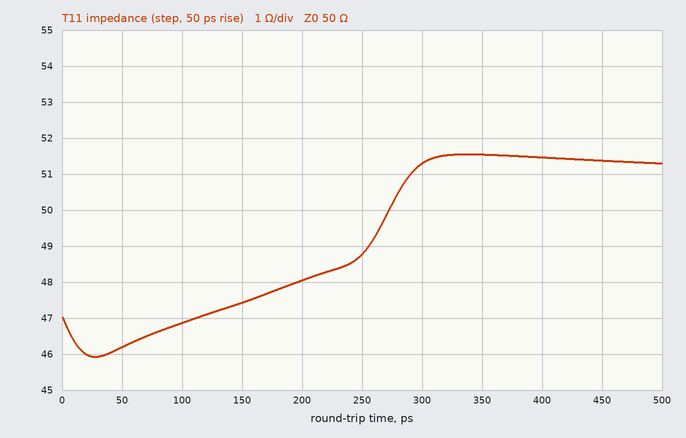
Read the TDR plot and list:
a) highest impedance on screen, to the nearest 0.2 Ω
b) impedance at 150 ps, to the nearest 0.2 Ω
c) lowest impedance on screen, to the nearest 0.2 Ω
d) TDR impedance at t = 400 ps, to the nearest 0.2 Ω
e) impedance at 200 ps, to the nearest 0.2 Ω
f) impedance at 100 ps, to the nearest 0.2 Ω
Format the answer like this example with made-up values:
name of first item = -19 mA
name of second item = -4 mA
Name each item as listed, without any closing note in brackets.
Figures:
highest impedance on screen, to the nearest 0.2 Ω = 51.6 Ω
impedance at 150 ps, to the nearest 0.2 Ω = 47.4 Ω
lowest impedance on screen, to the nearest 0.2 Ω = 46.0 Ω
TDR impedance at t = 400 ps, to the nearest 0.2 Ω = 51.4 Ω
impedance at 200 ps, to the nearest 0.2 Ω = 48.0 Ω
impedance at 100 ps, to the nearest 0.2 Ω = 46.8 Ω
